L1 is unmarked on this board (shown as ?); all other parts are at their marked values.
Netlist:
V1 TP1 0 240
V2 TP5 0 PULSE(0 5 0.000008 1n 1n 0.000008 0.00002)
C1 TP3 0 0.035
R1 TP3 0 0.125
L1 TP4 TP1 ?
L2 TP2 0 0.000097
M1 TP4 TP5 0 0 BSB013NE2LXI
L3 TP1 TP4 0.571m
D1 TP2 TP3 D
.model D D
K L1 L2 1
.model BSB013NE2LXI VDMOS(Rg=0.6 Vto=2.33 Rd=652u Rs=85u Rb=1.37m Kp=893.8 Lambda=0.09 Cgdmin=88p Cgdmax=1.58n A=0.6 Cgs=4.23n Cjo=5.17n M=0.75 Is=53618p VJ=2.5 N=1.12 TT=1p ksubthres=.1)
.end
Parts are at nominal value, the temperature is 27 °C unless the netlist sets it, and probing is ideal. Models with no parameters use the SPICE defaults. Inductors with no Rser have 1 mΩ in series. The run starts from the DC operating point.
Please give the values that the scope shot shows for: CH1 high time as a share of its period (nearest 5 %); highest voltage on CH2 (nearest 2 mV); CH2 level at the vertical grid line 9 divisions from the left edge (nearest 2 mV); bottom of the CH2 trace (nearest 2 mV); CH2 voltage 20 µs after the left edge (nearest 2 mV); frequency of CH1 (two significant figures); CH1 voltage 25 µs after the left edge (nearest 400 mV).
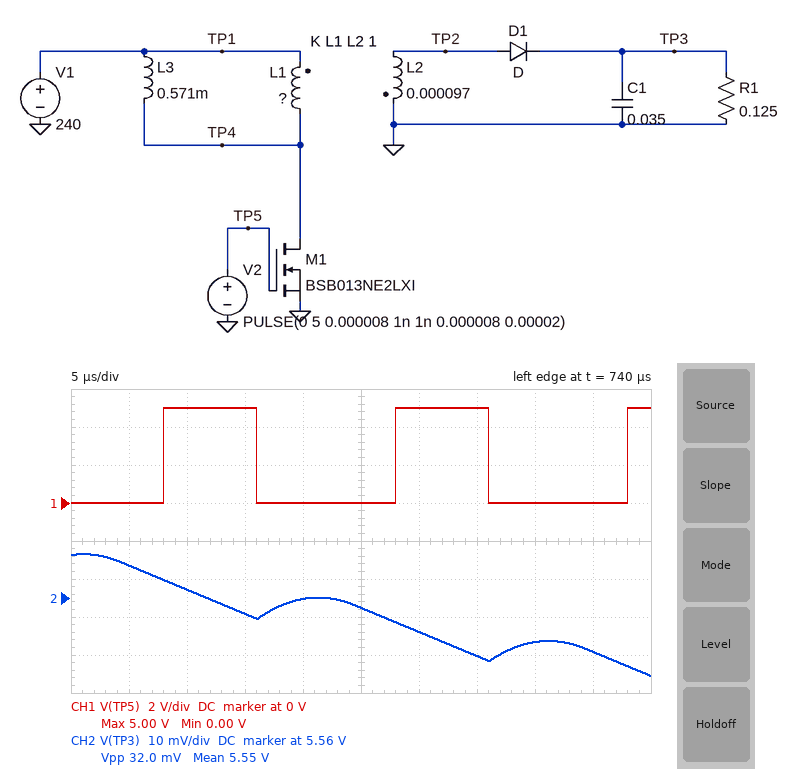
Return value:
40 %
5.572 V
5.546 V
5.540 V
5.560 V
50 kHz
0 V
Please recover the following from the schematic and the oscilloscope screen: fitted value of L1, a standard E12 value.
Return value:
120 mH
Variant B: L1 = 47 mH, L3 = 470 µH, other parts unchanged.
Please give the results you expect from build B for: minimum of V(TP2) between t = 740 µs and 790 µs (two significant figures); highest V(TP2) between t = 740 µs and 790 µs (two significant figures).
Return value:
-11 V
11 V
